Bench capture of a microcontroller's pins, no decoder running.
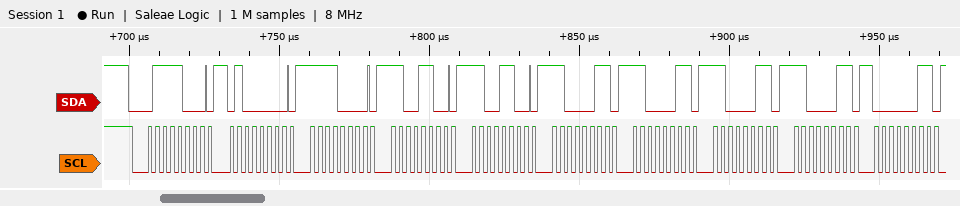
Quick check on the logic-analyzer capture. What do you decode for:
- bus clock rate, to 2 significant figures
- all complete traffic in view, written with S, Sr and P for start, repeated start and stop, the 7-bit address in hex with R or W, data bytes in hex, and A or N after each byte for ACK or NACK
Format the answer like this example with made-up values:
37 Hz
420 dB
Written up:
400 kHz
S 3CW A 40 A F0 A CC A CC A C3 A C3 A C3 A C3 A 03 A
